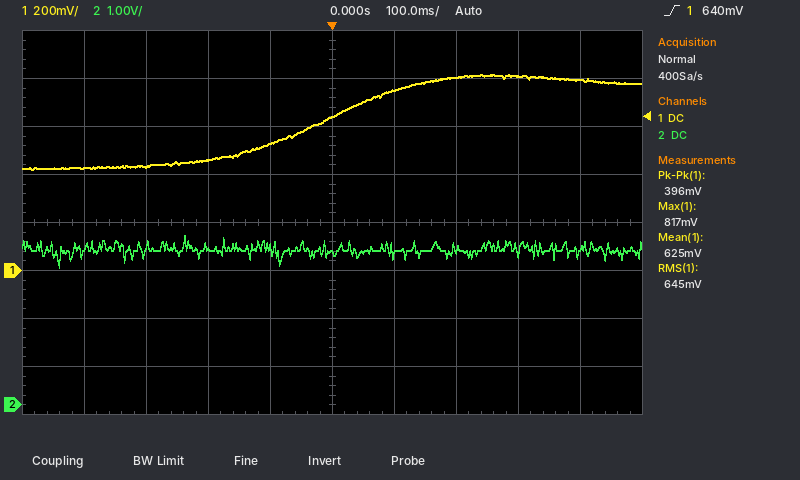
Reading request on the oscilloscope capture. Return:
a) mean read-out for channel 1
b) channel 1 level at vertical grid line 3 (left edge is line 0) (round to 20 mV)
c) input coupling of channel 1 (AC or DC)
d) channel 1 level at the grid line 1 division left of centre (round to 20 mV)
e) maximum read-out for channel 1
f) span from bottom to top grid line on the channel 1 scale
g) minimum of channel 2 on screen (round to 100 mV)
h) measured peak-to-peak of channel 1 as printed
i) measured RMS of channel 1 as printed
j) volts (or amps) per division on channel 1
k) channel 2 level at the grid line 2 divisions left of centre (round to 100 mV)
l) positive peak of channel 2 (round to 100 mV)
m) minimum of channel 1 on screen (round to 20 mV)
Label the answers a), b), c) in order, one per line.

a) 625 mV
b) 460 mV
c) DC
d) 520 mV
e) 817 mV
f) 1.6 V
g) 2.9 V
h) 396 mV
i) 645 mV
j) 200 mV
k) 3.3 V
l) 3.5 V
m) 420 mV
